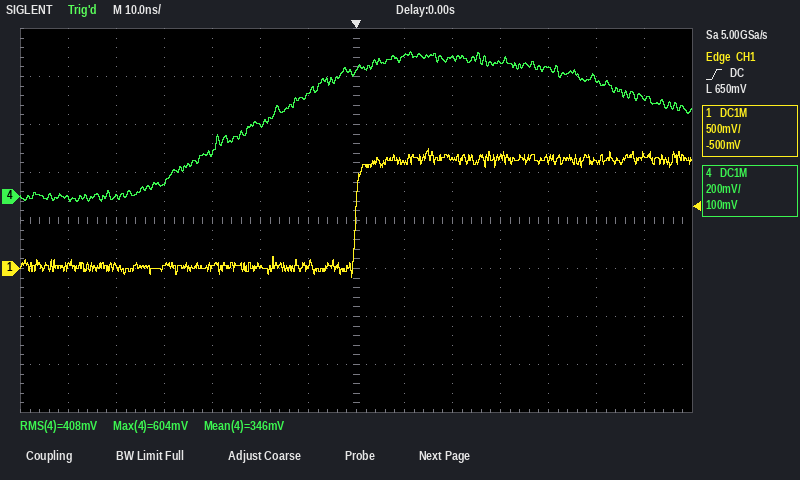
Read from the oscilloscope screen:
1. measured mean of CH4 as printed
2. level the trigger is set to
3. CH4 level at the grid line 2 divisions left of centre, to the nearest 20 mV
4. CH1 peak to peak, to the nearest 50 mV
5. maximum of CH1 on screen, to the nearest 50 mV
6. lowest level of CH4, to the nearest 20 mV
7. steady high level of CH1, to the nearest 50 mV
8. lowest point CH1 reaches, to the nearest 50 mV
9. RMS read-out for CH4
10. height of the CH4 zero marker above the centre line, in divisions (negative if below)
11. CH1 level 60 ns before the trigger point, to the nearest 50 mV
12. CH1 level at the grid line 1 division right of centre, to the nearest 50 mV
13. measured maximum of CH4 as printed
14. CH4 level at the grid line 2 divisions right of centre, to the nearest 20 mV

346 mV
650 mV
300 mV
1.35 V
1.25 V
-20 mV
1.15 V
-100 mV
408 mV
+0.5 div
0 mV
1.10 V
604 mV
580 mV
